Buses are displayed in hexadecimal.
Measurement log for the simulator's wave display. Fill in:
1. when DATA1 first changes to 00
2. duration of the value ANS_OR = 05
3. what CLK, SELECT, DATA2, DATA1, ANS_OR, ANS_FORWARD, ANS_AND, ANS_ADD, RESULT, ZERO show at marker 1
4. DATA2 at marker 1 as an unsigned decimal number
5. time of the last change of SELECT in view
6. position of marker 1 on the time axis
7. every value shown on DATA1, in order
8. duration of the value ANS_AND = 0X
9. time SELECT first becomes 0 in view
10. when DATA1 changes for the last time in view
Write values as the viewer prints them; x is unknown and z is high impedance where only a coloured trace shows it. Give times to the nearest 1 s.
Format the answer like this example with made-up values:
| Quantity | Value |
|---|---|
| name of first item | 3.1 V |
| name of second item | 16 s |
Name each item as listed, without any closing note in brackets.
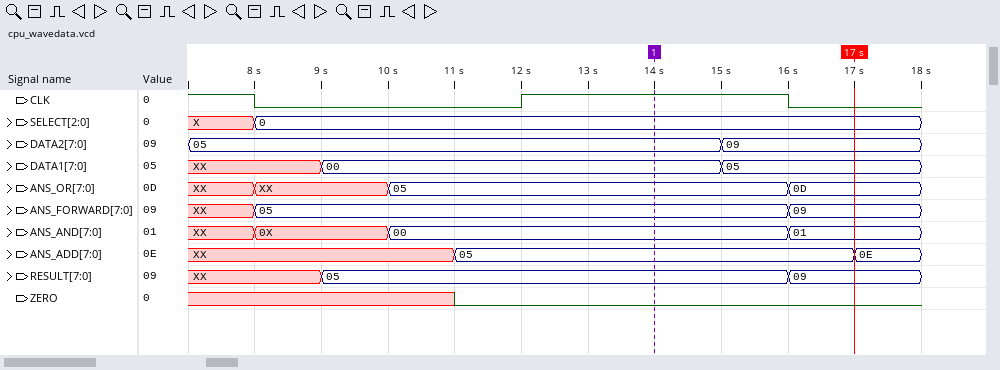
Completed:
| Quantity | Value |
|---|---|
| when DATA1 first changes to 00 | 9 s |
| duration of the value ANS_OR = 05 | 6 s |
| what CLK, SELECT, DATA2, DATA1, ANS_OR, ANS_FORWARD, ANS_AND, ANS_ADD, RESULT, ZERO show at marker 1 | CLK=1, SELECT=0, DATA2=05, DATA1=00, ANS_OR=05, ANS_FORWARD=05, ANS_AND=00, ANS_ADD=05, RESULT=05, ZERO=0 |
| DATA2 at marker 1 as an unsigned decimal number | 5 |
| time of the last change of SELECT in view | 8 s |
| position of marker 1 on the time axis | 14 s |
| every value shown on DATA1, in order | XX, 00, 05 |
| duration of the value ANS_AND = 0X | 2 s |
| time SELECT first becomes 0 in view | 8 s |
| when DATA1 changes for the last time in view | 15 s |
